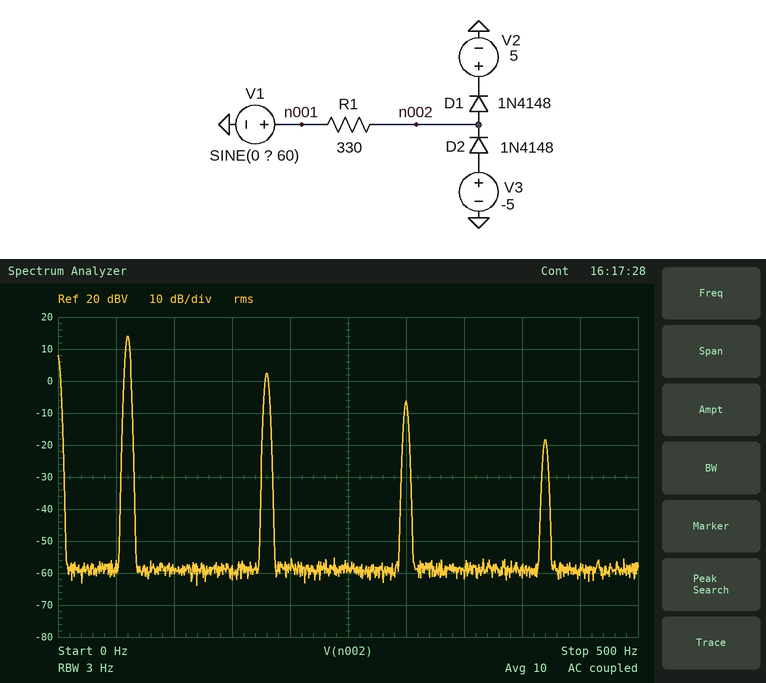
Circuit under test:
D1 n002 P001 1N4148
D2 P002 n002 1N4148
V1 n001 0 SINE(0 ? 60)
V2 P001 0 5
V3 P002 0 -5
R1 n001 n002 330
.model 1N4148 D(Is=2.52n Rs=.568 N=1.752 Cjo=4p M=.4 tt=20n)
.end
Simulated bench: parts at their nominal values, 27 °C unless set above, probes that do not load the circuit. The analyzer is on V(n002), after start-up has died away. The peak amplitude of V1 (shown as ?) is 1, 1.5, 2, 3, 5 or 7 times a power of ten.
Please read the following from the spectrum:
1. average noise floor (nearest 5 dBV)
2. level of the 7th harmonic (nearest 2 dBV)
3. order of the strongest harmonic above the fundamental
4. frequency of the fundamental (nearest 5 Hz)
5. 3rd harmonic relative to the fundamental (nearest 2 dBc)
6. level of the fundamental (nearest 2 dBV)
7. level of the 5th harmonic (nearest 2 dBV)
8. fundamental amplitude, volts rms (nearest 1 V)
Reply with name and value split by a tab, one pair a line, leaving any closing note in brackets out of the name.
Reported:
average noise floor	-60 dBV
level of the 7th harmonic	-18 dBV
order of the strongest harmonic above the fundamental	3
frequency of the fundamental	60 Hz
3rd harmonic relative to the fundamental	-12 dBc
level of the fundamental	14 dBV
level of the 5th harmonic	-6 dBV
fundamental amplitude, volts rms	5 V
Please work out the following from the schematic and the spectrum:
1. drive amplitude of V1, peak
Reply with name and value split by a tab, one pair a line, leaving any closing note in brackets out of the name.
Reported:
drive amplitude of V1, peak	15 V
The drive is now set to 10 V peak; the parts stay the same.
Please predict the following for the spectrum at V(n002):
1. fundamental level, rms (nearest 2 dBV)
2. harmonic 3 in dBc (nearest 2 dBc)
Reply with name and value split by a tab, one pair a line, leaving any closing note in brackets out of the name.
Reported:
fundamental level, rms	14 dBV
harmonic 3 in dBc	-14 dBc
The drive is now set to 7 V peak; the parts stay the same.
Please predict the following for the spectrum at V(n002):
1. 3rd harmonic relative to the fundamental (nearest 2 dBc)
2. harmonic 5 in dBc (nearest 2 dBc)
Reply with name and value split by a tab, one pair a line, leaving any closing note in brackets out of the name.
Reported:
3rd harmonic relative to the fundamental	-22 dBc
harmonic 5 in dBc	-30 dBc
